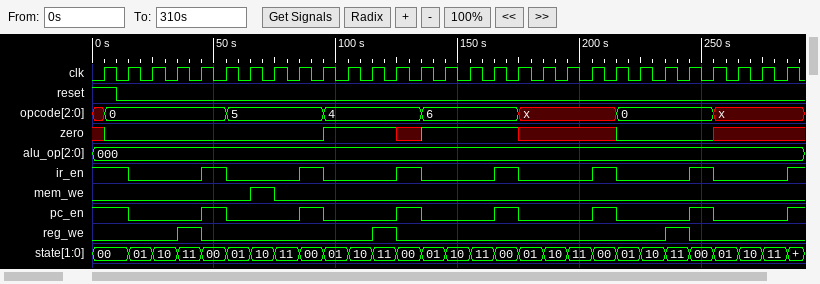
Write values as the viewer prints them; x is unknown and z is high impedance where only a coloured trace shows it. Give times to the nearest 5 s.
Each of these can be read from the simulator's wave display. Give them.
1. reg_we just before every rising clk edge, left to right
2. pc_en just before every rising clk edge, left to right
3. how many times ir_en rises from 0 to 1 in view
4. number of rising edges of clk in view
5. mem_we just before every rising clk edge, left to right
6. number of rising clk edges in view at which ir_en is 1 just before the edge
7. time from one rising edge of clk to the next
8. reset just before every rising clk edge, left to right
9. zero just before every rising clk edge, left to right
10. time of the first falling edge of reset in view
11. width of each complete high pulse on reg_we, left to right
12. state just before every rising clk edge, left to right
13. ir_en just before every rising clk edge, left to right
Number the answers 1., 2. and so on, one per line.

1. 0 0 0 0 1 0 0 0 0 0 0 0 1 0 0 0 0 0 0 0 0 0 0 0 1 0 0 0 0
2. 1 1 0 0 0 1 0 0 0 1 0 0 0 1 0 0 0 1 0 0 0 1 0 0 0 1 0 0 0
3. 7
4. 29
5. 0 0 0 0 0 0 0 1 0 0 0 0 0 0 0 0 0 0 0 0 0 0 0 0 0 0 0 0 0
6. 8
7. 10 s
8. 1 0 0 0 0 0 0 0 0 0 0 0 0 0 0 0 0 0 0 0 0 0 0 0 0 0 0 0 0
9. x 0 0 0 0 0 0 0 0 0 1 1 1 x 1 1 1 1 x x x x 0 0 0 0 x x x
10. 10 s
11. 10 s, 10 s, 10 s
12. 00, 00, 01, 10, 11, 00, 01, 10, 11, 00, 01, 10, 11, 00, 01, 10, 11, 00, 01, 10, 11, 00, 01, 10, 11, 00, 01, 10, 11
13. 1 1 0 0 0 1 0 0 0 1 0 0 0 1 0 0 0 1 0 0 0 1 0 0 0 1 0 0 0
